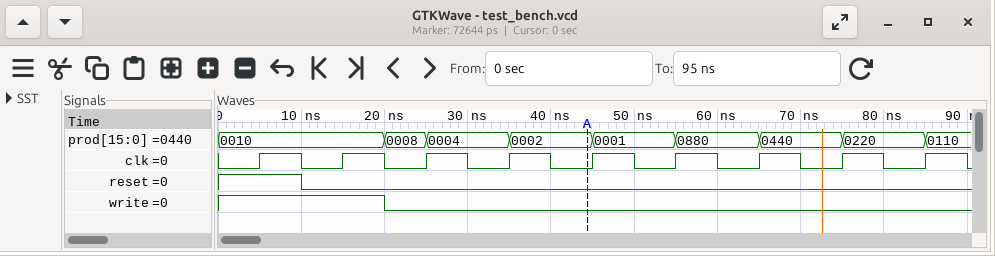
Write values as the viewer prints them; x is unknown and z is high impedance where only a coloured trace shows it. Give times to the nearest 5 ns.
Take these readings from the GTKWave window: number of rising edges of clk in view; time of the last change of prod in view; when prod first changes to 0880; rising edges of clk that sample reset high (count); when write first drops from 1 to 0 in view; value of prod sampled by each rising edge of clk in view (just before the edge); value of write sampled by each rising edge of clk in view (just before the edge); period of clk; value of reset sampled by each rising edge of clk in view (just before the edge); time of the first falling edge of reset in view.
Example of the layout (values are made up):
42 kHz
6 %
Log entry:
9
85 ns
55 ns
1
20 ns
0010, 0010, 0008, 0004, 0002, 0001, 0880, 0440, 0220
1 1 0 0 0 0 0 0 0
10 ns
1 0 0 0 0 0 0 0 0
10 ns
